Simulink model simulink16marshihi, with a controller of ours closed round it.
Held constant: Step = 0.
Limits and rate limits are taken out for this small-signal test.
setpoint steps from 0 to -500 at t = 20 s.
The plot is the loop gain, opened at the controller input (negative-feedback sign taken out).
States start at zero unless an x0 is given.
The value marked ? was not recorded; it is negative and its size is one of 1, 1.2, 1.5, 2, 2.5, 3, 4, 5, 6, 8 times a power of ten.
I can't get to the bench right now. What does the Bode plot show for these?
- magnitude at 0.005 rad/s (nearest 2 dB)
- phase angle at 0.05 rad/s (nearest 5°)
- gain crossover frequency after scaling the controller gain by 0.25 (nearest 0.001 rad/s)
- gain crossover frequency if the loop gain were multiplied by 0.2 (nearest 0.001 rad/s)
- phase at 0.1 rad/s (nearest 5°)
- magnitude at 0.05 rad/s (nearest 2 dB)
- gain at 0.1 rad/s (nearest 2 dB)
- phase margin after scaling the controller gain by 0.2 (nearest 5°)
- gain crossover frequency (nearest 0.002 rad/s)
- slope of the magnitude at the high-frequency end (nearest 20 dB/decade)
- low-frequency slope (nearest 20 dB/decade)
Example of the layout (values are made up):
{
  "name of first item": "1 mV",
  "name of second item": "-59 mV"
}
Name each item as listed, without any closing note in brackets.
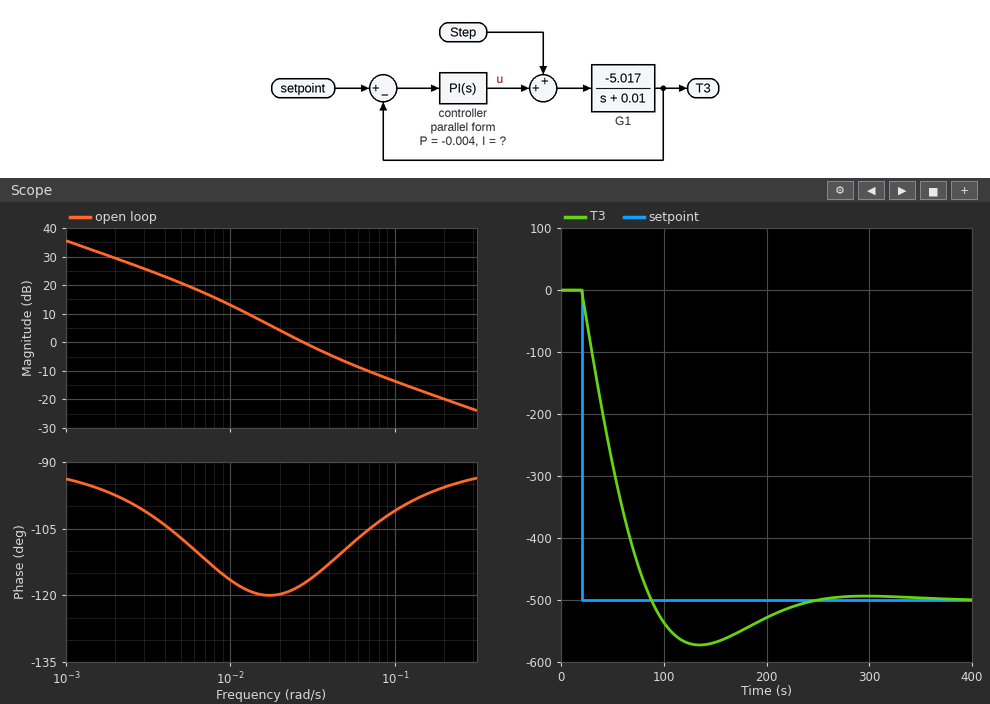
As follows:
{
  "magnitude at 0.005 rad/s": "20 dB",
  "phase angle at 0.05 rad/s": "-110°",
  "gain crossover frequency after scaling the controller gain by 0.25": "0.011 rad/s",
  "gain crossover frequency if the loop gain were multiplied by 0.2": "0.009 rad/s",
  "phase at 0.1 rad/s": "-100°",
  "magnitude at 0.05 rad/s": "-6 dB",
  "gain at 0.1 rad/s": "-14 dB",
  "phase margin after scaling the controller gain by 0.2": "65°",
  "gain crossover frequency": "0.028 rad/s",
  "slope of the magnitude at the high-frequency end": "-20 dB/decade",
  "low-frequency slope": "-20 dB/decade"
}
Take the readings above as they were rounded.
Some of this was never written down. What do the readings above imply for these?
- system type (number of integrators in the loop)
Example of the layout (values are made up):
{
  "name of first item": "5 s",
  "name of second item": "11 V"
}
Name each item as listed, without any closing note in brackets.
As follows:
{
  "system type": "1"
}
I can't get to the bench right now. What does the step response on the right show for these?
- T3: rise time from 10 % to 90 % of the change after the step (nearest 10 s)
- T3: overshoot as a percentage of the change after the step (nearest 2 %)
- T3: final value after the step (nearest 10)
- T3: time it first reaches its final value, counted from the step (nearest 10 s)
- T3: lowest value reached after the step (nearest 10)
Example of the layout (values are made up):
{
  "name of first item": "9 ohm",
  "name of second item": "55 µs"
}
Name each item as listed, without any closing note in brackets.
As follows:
{
  "T3: rise time from 10 % to 90 % of the change after the step": "50 s",
  "T3: overshoot as a percentage of the change after the step": "14 %",
  "T3: final value after the step": "-500",
  "T3: time it first reaches its final value, counted from the step": "70 s",
  "T3: lowest value reached after the step": "-570"
}
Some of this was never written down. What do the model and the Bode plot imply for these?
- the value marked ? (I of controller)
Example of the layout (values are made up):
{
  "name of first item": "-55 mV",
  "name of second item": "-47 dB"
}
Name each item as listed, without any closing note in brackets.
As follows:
{
  "the value marked ?": "-0.00012"
}
